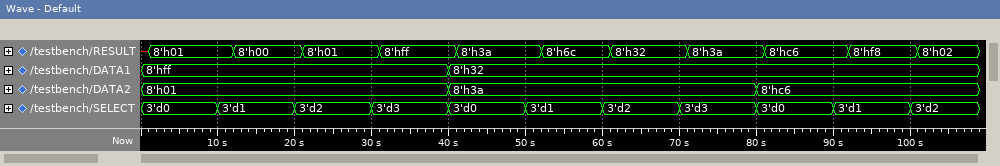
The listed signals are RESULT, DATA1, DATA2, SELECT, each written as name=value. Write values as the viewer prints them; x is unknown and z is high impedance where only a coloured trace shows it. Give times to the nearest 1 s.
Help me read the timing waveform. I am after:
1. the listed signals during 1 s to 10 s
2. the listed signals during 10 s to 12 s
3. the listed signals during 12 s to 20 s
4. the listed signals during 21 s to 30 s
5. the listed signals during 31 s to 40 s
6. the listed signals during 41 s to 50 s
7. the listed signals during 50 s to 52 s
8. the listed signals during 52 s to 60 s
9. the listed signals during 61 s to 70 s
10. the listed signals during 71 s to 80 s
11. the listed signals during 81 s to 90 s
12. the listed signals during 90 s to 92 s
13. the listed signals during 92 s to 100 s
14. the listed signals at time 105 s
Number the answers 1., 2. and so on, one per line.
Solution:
1. RESULT=8'h01, DATA1=8'hff, DATA2=8'h01, SELECT=3'd0
2. RESULT=8'h01, DATA1=8'hff, DATA2=8'h01, SELECT=3'd1
3. RESULT=8'h00, DATA1=8'hff, DATA2=8'h01, SELECT=3'd1
4. RESULT=8'h01, DATA1=8'hff, DATA2=8'h01, SELECT=3'd2
5. RESULT=8'hff, DATA1=8'hff, DATA2=8'h01, SELECT=3'd3
6. RESULT=8'h3a, DATA1=8'h32, DATA2=8'h3a, SELECT=3'd0
7. RESULT=8'h3a, DATA1=8'h32, DATA2=8'h3a, SELECT=3'd1
8. RESULT=8'h6c, DATA1=8'h32, DATA2=8'h3a, SELECT=3'd1
9. RESULT=8'h32, DATA1=8'h32, DATA2=8'h3a, SELECT=3'd2
10. RESULT=8'h3a, DATA1=8'h32, DATA2=8'h3a, SELECT=3'd3
11. RESULT=8'hc6, DATA1=8'h32, DATA2=8'hc6, SELECT=3'd0
12. RESULT=8'hc6, DATA1=8'h32, DATA2=8'hc6, SELECT=3'd1
13. RESULT=8'hf8, DATA1=8'h32, DATA2=8'hc6, SELECT=3'd1
14. RESULT=8'h02, DATA1=8'h32, DATA2=8'hc6, SELECT=3'd2
